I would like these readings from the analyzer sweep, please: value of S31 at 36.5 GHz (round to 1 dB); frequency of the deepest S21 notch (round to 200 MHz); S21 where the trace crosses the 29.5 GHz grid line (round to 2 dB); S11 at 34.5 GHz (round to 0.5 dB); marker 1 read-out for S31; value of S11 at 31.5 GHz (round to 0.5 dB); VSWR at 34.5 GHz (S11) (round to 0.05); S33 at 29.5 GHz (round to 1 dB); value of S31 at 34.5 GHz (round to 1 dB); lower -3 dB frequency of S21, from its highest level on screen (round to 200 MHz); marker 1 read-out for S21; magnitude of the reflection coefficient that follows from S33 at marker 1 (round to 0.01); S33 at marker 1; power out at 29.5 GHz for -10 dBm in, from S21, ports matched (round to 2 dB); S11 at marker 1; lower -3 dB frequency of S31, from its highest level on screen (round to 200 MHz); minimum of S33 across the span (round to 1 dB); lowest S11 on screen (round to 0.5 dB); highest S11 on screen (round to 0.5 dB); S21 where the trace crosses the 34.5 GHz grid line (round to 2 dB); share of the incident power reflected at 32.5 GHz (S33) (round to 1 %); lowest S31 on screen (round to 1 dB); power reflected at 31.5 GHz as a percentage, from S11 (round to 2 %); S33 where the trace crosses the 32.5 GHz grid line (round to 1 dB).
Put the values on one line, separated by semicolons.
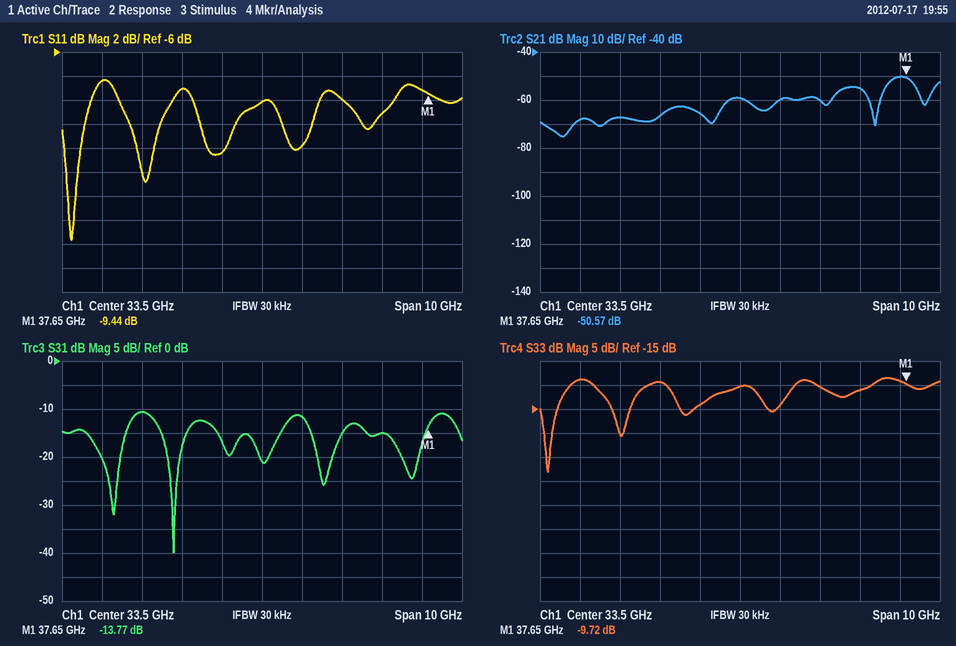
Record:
-15 dB; 29.0 GHz; -68 dB; -14.0 dB; -13.77 dB; -9.0 dB; 1.50; -9 dB; -12 dB; 37.2 GHz; -50.57 dB; 0.33; -9.72 dB; -78 dBm; -9.44 dB; 30.2 GHz; -28 dB; -21.5 dB; -8.5 dB; -60 dB; 4 %; -40 dB; 12 %; -14 dB
